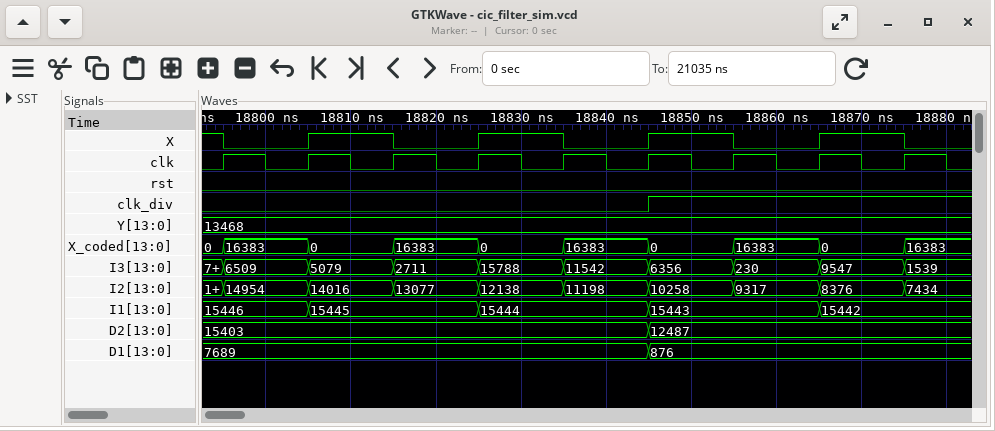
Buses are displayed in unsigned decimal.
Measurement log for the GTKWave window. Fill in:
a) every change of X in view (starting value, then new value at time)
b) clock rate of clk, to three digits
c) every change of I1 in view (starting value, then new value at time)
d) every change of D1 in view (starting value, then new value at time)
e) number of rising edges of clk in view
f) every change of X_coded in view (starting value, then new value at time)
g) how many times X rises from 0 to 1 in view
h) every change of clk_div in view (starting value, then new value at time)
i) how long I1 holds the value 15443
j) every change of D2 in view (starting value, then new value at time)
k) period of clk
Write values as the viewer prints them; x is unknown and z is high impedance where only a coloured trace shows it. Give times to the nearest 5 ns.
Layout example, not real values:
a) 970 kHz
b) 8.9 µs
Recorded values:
a) 1, 0 at 18795 ns, 1 at 18805 ns, 0 at 18815 ns, 1 at 18825 ns, 0 at 18835 ns, 1 at 18845 ns, 0 at 18855 ns, 1 at 18865 ns, 0 at 18875 ns
b) 100 MHz
c) 15446, 15445 at 18805 ns, 15444 at 18825 ns, 15443 at 18845 ns, 15442 at 18865 ns
d) 7689, 876 at 18845 ns
e) 9
f) 0, 16383 at 18795 ns, 0 at 18805 ns, 16383 at 18815 ns, 0 at 18825 ns, 16383 at 18835 ns, 0 at 18845 ns, 16383 at 18855 ns, 0 at 18865 ns, 16383 at 18875 ns
g) 4
h) 0, 1 at 18845 ns
i) 20 ns
j) 15403, 12487 at 18845 ns
k) 10 ns
